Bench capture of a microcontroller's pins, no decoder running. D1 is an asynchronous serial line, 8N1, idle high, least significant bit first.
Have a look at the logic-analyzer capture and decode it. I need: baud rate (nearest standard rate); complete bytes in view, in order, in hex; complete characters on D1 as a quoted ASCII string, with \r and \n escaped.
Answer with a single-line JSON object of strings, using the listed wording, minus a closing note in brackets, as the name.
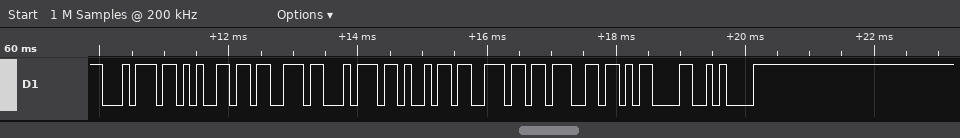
{"baud rate": "9600 baud", "complete bytes in view, in order, in hex": "0x74 0x65 0x73 0x74 0x69 0x6E 0x67 0x0D 0x0A", "complete characters on D1 as a quoted ASCII string, with \\r and \\n escaped": "\"testing\\r\\n\""}
